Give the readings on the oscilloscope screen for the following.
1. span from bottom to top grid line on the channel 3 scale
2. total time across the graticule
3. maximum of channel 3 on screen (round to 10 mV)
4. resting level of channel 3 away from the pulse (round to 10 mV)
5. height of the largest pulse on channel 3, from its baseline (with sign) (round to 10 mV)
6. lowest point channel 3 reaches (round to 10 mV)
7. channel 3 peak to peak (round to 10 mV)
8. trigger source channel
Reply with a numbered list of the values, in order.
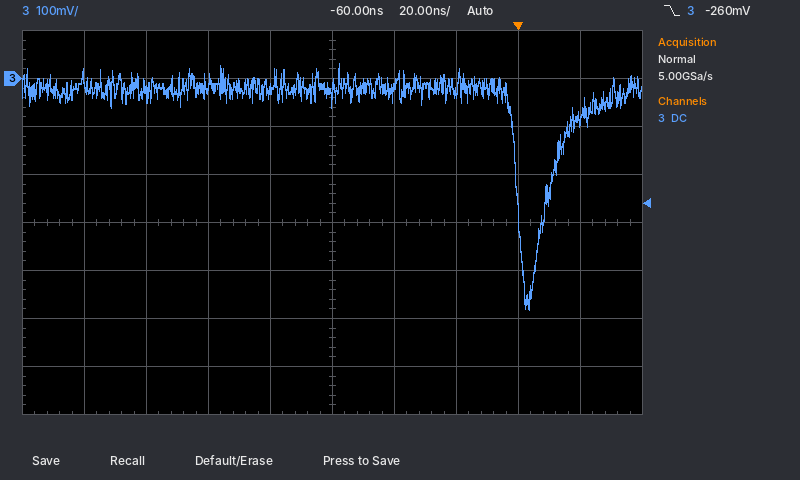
1. 800 mV
2. 200 ns
3. 30 mV
4. -20 mV
5. -460 mV
6. -480 mV
7. 510 mV
8. channel 3
